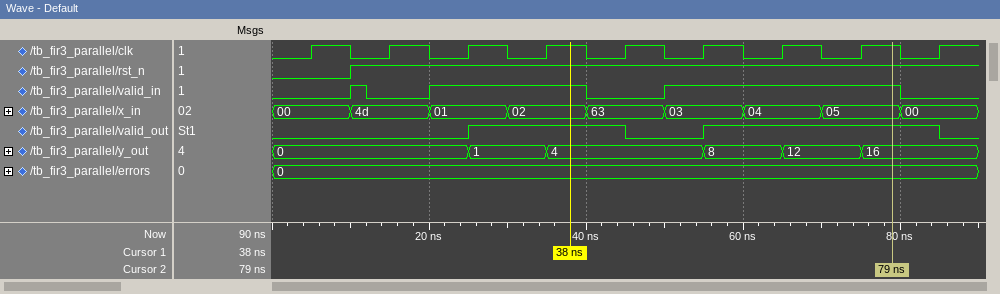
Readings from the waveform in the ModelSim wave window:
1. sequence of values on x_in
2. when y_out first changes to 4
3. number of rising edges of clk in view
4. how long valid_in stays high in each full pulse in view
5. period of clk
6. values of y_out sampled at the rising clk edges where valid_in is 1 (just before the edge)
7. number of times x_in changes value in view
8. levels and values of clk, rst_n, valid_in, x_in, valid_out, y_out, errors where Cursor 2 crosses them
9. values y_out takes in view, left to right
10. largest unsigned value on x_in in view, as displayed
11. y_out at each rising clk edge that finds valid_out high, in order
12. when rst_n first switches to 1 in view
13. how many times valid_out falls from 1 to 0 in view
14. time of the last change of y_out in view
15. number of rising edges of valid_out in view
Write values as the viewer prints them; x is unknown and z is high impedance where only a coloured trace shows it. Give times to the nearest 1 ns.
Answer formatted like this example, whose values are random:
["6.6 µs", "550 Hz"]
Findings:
["00, 4d, 01, 02, 63, 03, 04, 05, 00", "35 ns", "9", "2 ns, 20 ns, 30 ns", "10 ns", "0, 1, 4, 8, 12", "8", "clk=1, rst_n=1, valid_in=1, x_in=05, valid_out=1, y_out=16, errors=0", "0, 1, 4, 8, 12, 16", "63", "1, 4, 8, 12, 16", "10 ns", "2", "75 ns", "2"]
